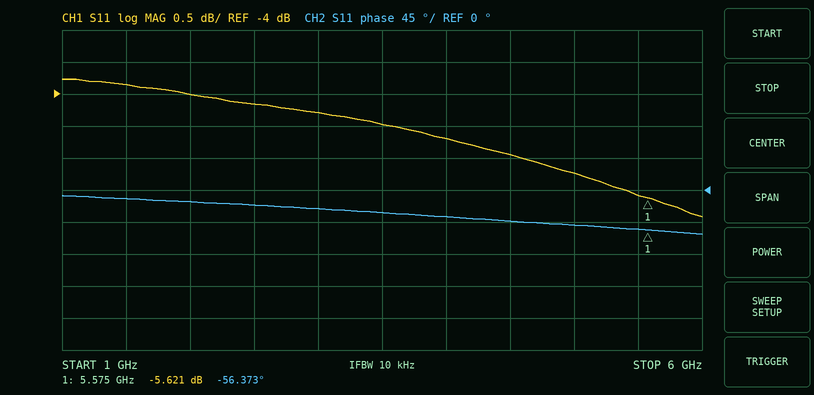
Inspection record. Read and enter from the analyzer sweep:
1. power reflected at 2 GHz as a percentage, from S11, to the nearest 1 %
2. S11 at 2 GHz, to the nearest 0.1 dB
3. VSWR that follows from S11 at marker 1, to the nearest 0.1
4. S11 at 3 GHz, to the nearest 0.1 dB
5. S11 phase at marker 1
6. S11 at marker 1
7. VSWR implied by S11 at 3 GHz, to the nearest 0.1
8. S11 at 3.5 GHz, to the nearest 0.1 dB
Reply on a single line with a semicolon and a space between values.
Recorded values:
40 %; -4.0 dB; 3.2; -4.3 dB; -56.373°; -5.621 dB; 4.1; -4.5 dB
